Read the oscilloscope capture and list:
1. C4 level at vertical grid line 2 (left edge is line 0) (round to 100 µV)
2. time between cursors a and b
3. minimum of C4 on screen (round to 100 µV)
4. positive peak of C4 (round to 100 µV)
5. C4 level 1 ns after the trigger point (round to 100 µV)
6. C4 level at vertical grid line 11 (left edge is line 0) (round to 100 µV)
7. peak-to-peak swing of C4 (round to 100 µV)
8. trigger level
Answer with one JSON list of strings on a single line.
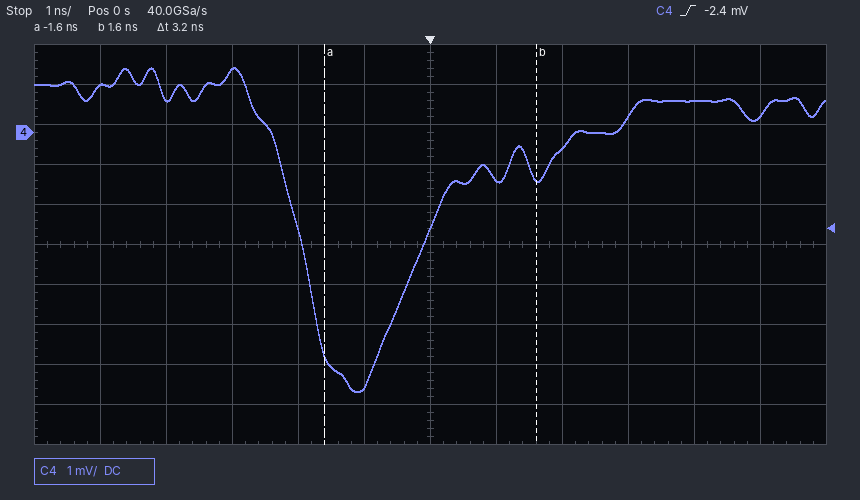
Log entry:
["900 µV", "3.2 ns", "-6.5 mV", "1.6 mV", "-1.2 mV", "400 µV", "8.1 mV", "-2.4 mV"]
